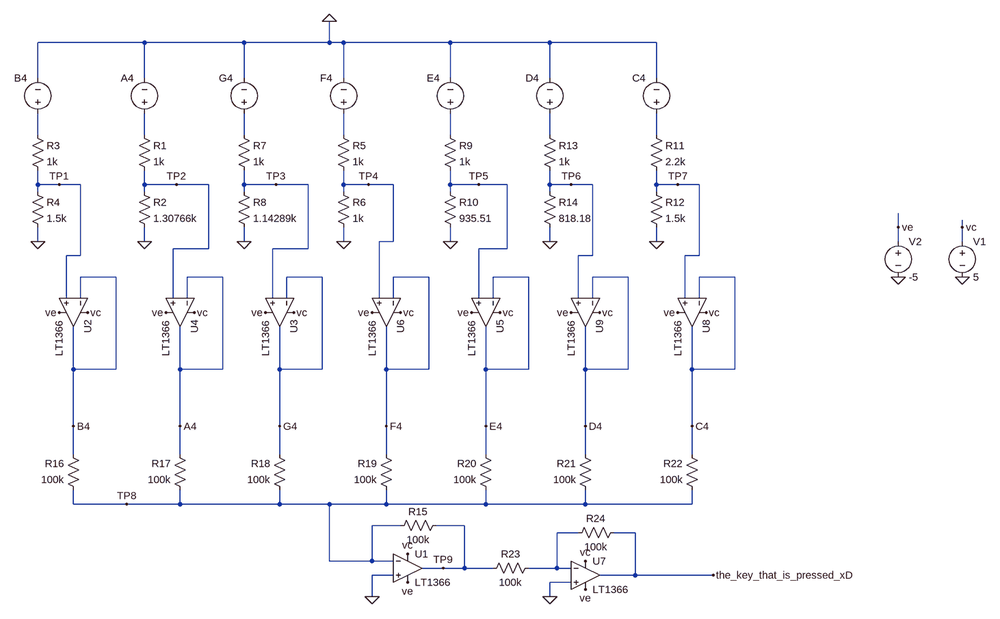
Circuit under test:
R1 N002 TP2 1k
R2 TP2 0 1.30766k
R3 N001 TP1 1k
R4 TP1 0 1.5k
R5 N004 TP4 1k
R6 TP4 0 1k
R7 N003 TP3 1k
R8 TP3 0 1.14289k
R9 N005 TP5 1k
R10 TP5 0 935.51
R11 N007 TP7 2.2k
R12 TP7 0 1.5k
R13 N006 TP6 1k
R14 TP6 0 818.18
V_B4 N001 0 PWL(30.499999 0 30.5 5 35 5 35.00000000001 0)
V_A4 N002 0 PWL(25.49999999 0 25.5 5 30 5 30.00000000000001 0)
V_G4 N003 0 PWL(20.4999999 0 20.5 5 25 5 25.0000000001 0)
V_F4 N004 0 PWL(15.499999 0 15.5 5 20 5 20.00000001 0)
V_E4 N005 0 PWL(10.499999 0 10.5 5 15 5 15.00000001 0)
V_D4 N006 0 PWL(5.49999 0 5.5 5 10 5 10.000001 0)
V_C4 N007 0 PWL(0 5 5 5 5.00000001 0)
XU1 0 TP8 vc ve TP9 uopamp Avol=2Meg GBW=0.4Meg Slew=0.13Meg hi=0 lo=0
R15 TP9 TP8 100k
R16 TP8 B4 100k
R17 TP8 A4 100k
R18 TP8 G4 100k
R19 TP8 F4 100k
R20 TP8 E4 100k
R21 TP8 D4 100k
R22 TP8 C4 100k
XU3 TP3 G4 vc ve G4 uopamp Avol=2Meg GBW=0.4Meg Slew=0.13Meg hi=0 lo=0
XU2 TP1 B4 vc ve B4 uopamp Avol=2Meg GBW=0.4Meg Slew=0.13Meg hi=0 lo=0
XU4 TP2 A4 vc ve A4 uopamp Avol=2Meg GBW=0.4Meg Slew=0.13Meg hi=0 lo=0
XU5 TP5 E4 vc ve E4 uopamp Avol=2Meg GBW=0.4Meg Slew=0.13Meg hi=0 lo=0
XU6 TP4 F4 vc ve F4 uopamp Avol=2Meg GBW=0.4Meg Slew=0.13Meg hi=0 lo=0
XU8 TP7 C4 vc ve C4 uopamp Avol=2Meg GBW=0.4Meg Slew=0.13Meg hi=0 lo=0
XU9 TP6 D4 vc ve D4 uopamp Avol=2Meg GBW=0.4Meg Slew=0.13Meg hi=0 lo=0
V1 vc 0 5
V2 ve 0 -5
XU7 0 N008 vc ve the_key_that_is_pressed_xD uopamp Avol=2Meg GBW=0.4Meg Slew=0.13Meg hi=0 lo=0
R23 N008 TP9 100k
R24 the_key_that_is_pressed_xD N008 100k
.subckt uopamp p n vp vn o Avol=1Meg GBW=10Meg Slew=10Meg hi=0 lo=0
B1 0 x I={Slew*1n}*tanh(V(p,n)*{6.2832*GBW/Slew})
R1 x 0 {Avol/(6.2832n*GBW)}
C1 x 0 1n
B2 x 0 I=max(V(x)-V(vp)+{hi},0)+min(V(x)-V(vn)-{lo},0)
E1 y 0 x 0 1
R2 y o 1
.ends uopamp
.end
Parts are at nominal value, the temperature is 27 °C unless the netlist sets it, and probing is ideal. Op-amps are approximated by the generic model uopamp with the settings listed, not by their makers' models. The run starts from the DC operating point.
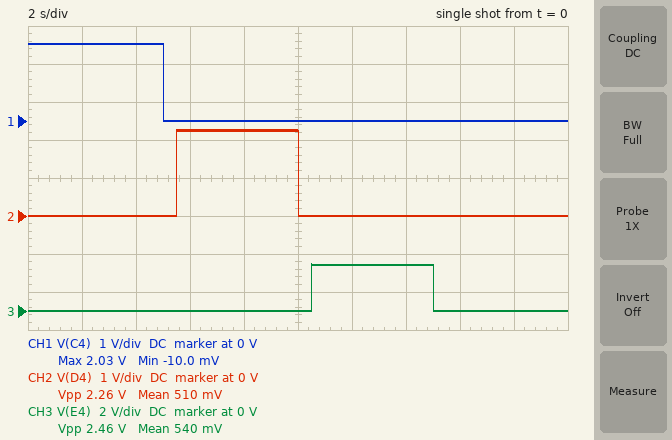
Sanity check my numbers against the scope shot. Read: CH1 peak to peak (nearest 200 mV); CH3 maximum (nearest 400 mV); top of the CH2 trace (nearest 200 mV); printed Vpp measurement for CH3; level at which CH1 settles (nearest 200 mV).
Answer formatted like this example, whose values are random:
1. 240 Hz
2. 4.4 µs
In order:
1. 2.0 V
2. 2.4 V
3. 2.2 V
4. 2.46 V
5. 0 V
